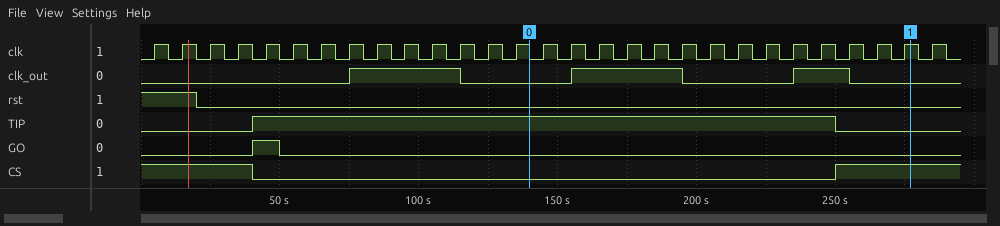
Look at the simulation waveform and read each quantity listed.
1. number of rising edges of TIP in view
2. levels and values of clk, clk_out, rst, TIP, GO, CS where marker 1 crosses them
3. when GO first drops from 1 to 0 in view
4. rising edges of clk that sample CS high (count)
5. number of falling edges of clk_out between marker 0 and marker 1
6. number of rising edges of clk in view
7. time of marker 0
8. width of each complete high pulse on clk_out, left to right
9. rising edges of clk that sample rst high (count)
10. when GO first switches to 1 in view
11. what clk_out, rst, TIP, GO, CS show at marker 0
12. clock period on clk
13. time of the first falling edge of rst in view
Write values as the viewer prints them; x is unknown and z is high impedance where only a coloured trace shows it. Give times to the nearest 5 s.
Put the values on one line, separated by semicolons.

1; clk=1, clk_out=0, rst=0, TIP=0, GO=0, CS=1; 50 s; 8; 2; 29; 140 s; 40 s, 40 s, 20 s; 2; 40 s; clk_out=0, rst=0, TIP=1, GO=0, CS=0; 10 s; 20 s
